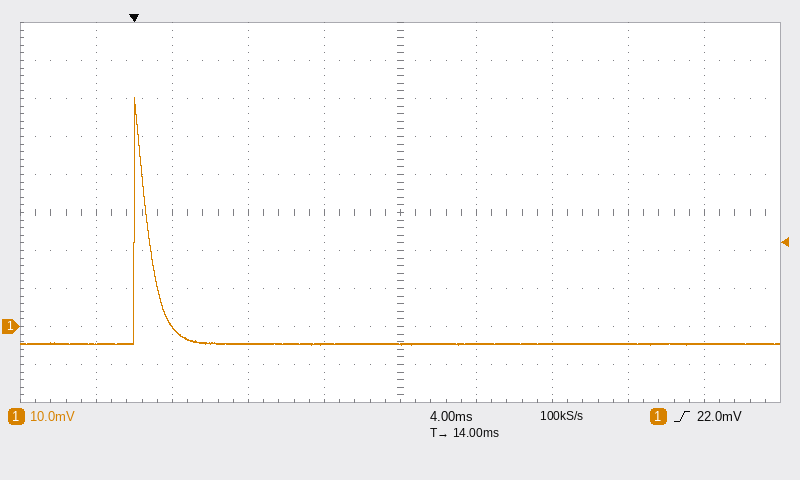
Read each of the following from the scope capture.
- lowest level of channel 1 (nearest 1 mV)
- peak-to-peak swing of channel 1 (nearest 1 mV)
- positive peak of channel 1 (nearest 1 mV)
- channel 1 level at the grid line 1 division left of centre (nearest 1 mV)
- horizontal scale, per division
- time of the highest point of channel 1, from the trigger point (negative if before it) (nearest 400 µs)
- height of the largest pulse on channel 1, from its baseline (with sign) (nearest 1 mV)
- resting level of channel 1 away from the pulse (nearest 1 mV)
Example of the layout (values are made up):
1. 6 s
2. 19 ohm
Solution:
1. -5 mV
2. 65 mV
3. 60 mV
4. -5 mV
5. 4 ms
6. 0.0 ms
7. +65 mV
8. -5 mV
